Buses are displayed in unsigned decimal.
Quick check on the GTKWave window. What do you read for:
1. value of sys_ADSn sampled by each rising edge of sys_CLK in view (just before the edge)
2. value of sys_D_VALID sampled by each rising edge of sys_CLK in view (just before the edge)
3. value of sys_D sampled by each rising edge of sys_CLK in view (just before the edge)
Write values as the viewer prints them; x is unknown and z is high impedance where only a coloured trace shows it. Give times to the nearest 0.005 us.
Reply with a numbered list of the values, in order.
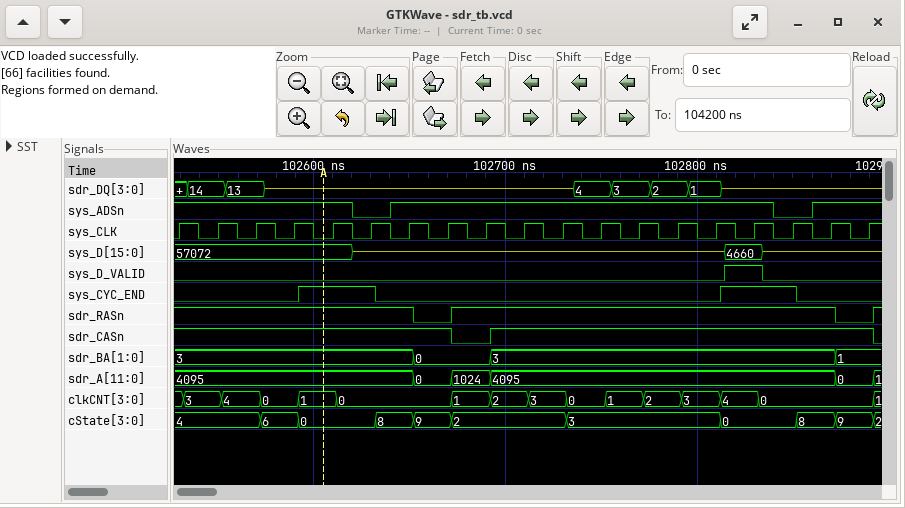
1. 1 1 1 1 1 0 1 1 1 1 1 1 1 1 1 1 0 1 1
2. 0 0 0 0 0 0 0 0 0 0 0 0 0 0 0 1 0 0 0
3. 57072, 57072, 57072, 57072, 57072, z, z, z, z, z, z, z, z, z, z, 4660, z, z, z
